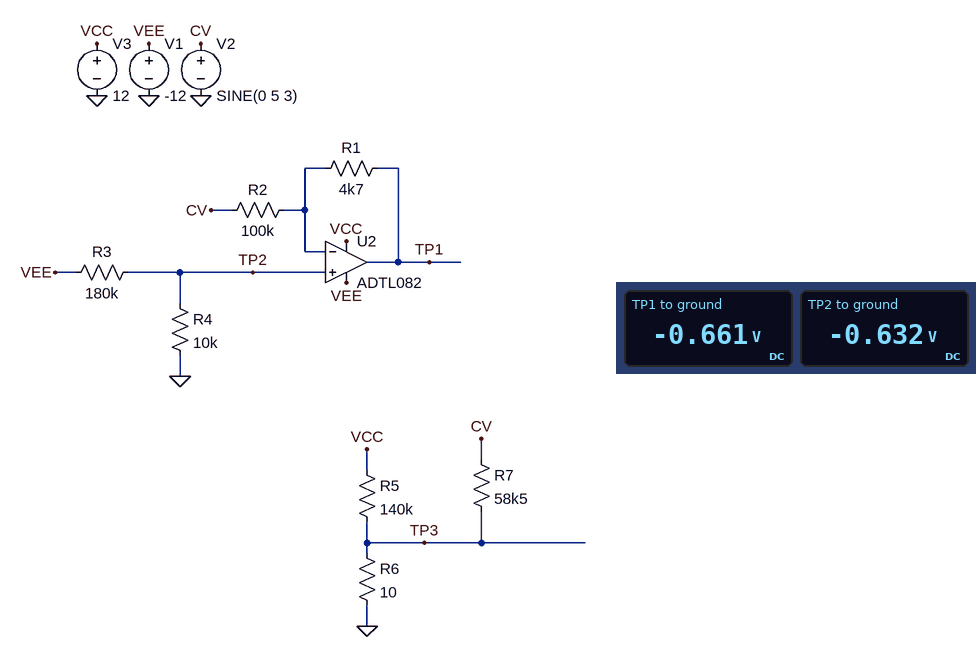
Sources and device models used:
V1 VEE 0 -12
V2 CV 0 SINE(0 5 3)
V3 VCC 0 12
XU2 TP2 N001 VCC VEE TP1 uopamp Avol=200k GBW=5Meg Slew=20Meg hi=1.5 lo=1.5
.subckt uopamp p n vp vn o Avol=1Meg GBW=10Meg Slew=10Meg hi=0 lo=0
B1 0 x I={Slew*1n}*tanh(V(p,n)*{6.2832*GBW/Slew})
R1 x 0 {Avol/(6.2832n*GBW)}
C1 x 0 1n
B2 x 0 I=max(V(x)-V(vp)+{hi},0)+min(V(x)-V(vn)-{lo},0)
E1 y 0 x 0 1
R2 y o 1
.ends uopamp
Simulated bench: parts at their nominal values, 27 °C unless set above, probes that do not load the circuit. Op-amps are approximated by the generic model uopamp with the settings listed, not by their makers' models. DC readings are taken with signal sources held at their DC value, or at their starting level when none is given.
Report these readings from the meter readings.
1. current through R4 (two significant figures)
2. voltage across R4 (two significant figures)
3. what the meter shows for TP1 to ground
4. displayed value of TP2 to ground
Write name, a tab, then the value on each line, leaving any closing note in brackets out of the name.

current through R4	63 µA
voltage across R4	630 mV
what the meter shows for TP1 to ground	-0.661 V
displayed value of TP2 to ground	-0.632 V
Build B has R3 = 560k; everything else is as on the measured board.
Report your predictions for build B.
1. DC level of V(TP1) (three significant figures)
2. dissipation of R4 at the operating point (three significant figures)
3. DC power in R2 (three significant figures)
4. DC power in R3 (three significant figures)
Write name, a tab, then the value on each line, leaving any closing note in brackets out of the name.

DC level of V(TP1)	-220 mV
dissipation of R4 at the operating point	4.43 µW
DC power in R2	443 nW
DC power in R3	248 µW
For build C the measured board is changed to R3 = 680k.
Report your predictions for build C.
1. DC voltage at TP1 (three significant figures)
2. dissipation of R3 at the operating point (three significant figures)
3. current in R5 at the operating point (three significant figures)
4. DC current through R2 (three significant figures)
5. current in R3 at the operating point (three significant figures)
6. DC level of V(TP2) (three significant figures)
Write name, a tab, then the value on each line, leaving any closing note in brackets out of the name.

DC voltage at TP1	-182 mV
dissipation of R3 at the operating point	206 µW
current in R5 at the operating point	85.7 µA
DC current through R2	1.74 µA
current in R3 at the operating point	17.4 µA
DC level of V(TP2)	-174 mV
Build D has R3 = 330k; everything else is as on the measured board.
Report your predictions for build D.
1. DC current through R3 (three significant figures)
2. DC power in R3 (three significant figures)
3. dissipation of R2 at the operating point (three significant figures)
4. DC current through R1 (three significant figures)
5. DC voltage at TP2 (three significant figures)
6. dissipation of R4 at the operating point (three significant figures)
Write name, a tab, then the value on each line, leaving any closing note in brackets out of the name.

DC current through R3	35.3 µA
DC power in R3	411 µW
dissipation of R2 at the operating point	1.25 µW
DC current through R1	3.53 µA
DC voltage at TP2	-353 mV
dissipation of R4 at the operating point	12.5 µW
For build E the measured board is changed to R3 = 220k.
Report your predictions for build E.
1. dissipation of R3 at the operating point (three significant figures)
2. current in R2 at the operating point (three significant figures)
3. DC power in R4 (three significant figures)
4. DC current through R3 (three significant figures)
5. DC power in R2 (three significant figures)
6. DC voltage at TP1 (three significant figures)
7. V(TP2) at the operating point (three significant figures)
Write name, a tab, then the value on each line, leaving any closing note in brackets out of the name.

dissipation of R3 at the operating point	599 µW
current in R2 at the operating point	5.22 µA
DC power in R4	27.2 µW
DC current through R3	52.2 µA
DC power in R2	2.72 µW
DC voltage at TP1	-546 mV
V(TP2) at the operating point	-522 mV
